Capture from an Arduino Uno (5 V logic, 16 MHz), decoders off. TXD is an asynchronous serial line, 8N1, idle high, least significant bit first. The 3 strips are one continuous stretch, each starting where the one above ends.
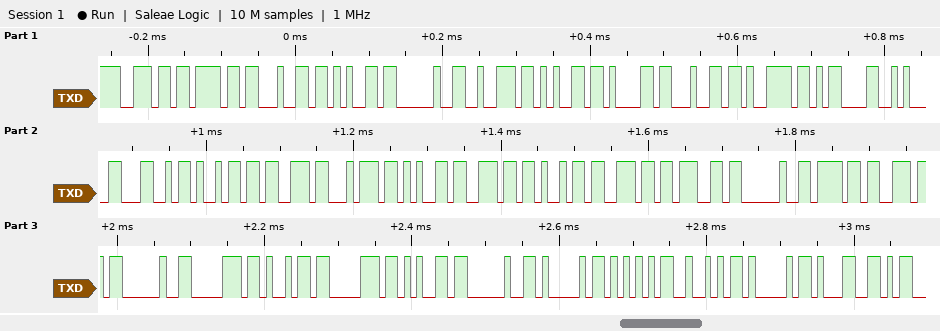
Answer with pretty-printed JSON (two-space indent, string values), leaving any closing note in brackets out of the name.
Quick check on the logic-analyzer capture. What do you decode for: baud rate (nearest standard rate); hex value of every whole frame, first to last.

{
  "baud rate": "115200 baud",
  "hex value of every whole frame, first to last": "6E 6F 64 65 20 72 65 61 64 79 0D 0A 4C 69 73 74 65 6E 69 6E 67 20 6F 6E 20 70 69 70 65 20 41 55 52 41 31"
}
